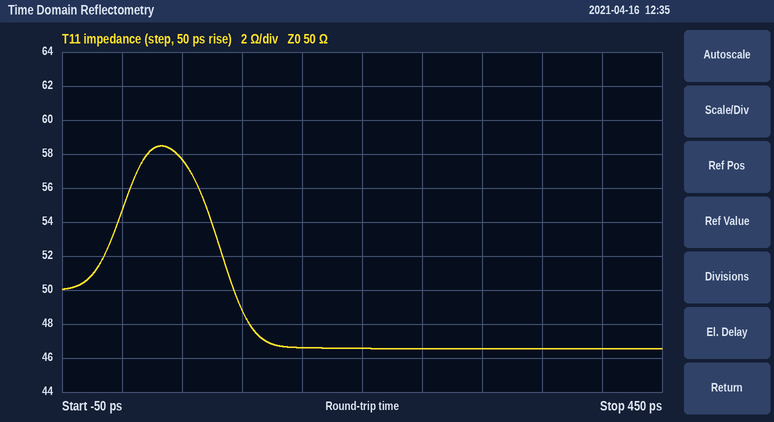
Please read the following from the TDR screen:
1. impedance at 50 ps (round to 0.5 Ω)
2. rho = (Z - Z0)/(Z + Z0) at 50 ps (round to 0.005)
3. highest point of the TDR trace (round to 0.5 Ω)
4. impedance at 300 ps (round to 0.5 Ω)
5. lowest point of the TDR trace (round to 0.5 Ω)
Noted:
57.5 Ω
+0.070
58.5 Ω
46.5 Ω
46.5 Ω
